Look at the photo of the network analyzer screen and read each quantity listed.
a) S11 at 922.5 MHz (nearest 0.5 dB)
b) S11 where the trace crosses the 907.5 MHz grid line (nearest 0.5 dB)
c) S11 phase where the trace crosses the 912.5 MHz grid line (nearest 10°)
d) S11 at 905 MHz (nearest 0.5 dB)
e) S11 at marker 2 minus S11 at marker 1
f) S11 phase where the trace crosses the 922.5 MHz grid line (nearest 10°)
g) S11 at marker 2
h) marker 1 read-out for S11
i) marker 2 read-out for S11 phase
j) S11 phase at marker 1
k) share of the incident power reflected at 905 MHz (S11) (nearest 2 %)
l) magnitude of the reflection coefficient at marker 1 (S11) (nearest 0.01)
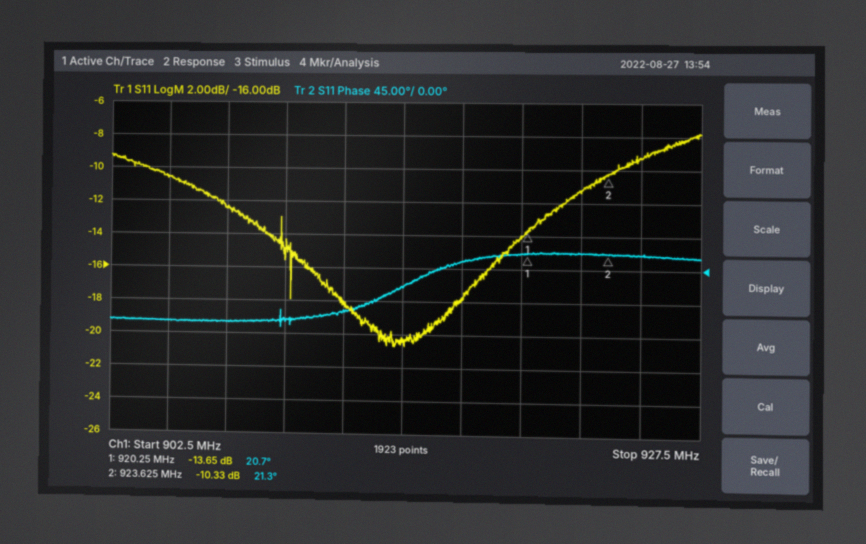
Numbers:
-11.5 dB
-12.5 dB
-60°
-10.5 dB
3.32 dB
20°
-10.33 dB
-13.65 dB
21.3°
20.7°
8 %
0.21
